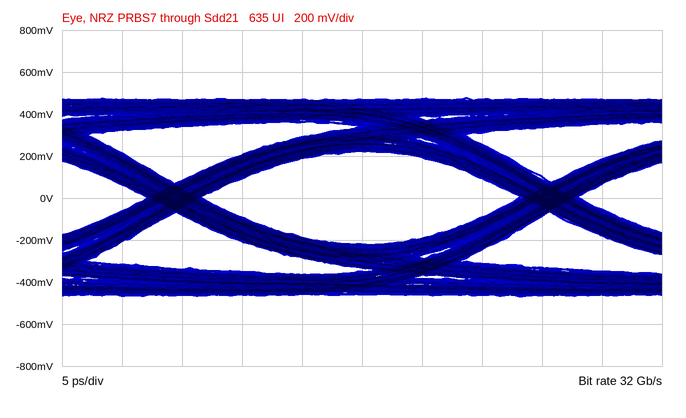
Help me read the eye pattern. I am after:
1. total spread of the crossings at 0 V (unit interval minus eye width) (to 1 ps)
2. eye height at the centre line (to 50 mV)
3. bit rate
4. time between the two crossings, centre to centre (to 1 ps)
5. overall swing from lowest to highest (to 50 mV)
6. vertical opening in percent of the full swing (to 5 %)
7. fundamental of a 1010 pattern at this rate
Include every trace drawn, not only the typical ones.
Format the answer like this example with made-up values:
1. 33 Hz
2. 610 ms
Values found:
1. 5 ps
2. 450 mV
3. 32 Gb/s
4. 31 ps
5. 950 mV
6. 45 %
7. 16 GHz
